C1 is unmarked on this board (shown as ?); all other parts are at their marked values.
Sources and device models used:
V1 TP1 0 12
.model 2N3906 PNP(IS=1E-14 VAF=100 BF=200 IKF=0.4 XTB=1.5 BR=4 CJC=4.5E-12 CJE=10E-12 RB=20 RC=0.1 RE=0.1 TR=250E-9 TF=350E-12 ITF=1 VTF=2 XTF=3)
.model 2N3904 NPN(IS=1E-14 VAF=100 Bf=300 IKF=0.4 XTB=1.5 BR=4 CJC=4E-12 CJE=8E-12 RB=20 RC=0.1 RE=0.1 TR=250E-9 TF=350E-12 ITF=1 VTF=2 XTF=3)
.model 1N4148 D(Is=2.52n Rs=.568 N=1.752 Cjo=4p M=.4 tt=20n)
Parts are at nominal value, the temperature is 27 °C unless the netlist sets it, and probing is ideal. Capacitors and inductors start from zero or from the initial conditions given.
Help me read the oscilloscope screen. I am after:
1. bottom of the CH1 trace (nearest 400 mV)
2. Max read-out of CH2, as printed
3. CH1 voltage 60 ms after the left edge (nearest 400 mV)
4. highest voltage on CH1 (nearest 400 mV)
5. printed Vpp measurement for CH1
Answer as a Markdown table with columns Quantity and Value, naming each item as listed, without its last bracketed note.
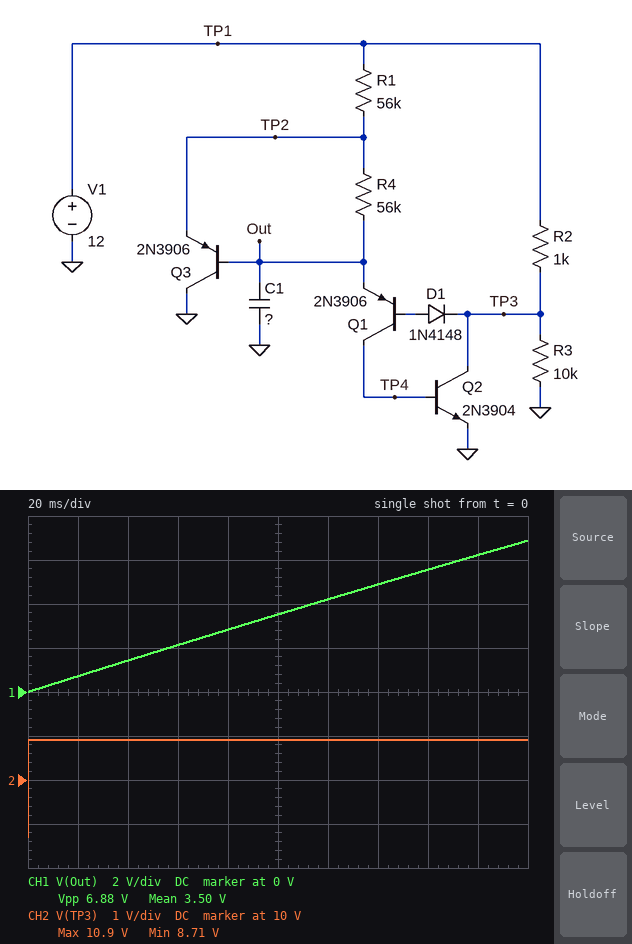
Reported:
| Quantity | Value |
|---|---|
| bottom of the CH1 trace | 0 V |
| Max read-out of CH2, as printed | 10.9 V |
| CH1 voltage 60 ms after the left edge | 2.0 V |
| highest voltage on CH1 | 6.8 V |
| printed Vpp measurement for CH1 | 6.88 V |
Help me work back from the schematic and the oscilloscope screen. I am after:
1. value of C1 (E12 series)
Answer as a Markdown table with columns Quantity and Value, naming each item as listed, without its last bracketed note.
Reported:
| Quantity | Value |
|---|---|
| value of C1 | 330 nF |
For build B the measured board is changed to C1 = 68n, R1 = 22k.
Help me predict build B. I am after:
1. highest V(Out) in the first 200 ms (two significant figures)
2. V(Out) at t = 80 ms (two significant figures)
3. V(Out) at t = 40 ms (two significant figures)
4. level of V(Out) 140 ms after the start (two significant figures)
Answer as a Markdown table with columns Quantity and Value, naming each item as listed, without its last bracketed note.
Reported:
| Quantity | Value |
|---|---|
| highest V(Out) in the first 200 ms | 11 V |
| V(Out) at t = 80 ms | 3.8 V |
| V(Out) at t = 40 ms | 7.5 V |
| level of V(Out) 140 ms after the start | 3.6 V |
